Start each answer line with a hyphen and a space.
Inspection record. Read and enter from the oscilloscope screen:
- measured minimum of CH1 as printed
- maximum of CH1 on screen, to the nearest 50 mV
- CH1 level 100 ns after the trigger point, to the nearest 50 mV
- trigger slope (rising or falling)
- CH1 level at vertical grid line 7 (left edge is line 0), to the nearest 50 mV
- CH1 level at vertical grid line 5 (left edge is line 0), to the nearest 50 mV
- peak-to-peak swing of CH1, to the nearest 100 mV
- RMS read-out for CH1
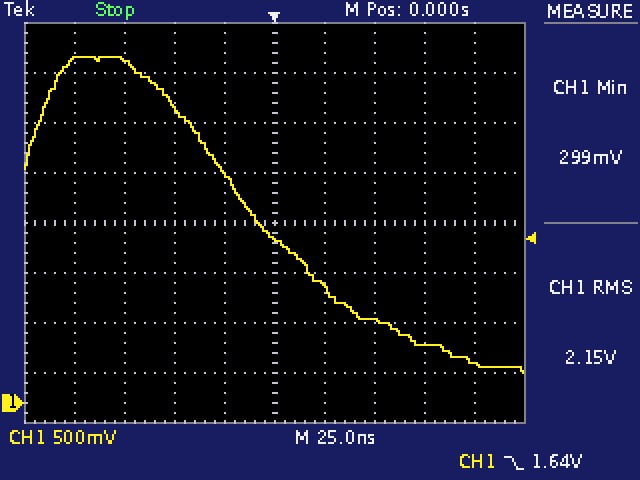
- 299 mV
- 3.45 V
- 400 mV
- falling
- 850 mV
- 1.65 V
- 3.20 V
- 2.15 V
